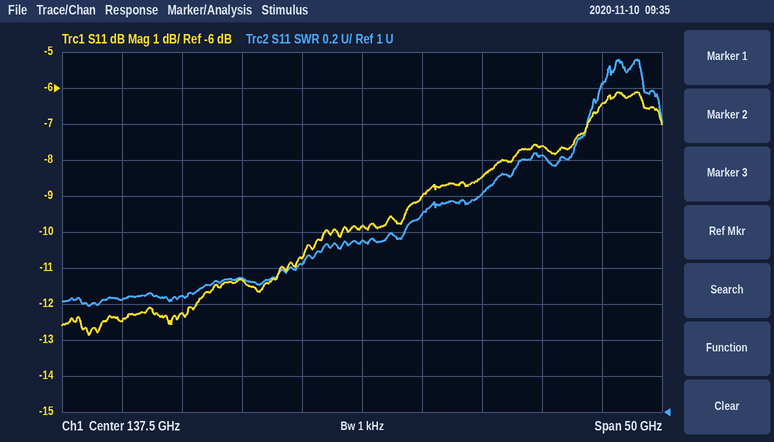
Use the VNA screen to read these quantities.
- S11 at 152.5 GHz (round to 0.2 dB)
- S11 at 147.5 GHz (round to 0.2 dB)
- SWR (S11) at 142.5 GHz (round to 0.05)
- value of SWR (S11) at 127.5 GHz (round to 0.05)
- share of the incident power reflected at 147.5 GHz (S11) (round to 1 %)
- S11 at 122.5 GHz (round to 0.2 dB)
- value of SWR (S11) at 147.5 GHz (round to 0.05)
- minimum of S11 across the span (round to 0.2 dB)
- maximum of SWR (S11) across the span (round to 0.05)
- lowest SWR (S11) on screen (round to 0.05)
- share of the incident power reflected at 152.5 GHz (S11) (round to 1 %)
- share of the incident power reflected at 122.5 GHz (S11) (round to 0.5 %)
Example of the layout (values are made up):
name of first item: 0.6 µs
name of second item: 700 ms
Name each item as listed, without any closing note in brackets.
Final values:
S11 at 152.5 GHz: -7.6 dB
S11 at 147.5 GHz: -8.4 dB
SWR (S11) at 142.5 GHz: 2.10
value of SWR (S11) at 127.5 GHz: 1.75
share of the incident power reflected at 147.5 GHz (S11): 14 %
S11 at 122.5 GHz: -12.2 dB
value of SWR (S11) at 147.5 GHz: 2.20
minimum of S11 across the span: -12.8 dB
maximum of SWR (S11) across the span: 2.95
lowest SWR (S11) on screen: 1.60
share of the incident power reflected at 152.5 GHz (S11): 17 %
share of the incident power reflected at 122.5 GHz (S11): 6.0 %
